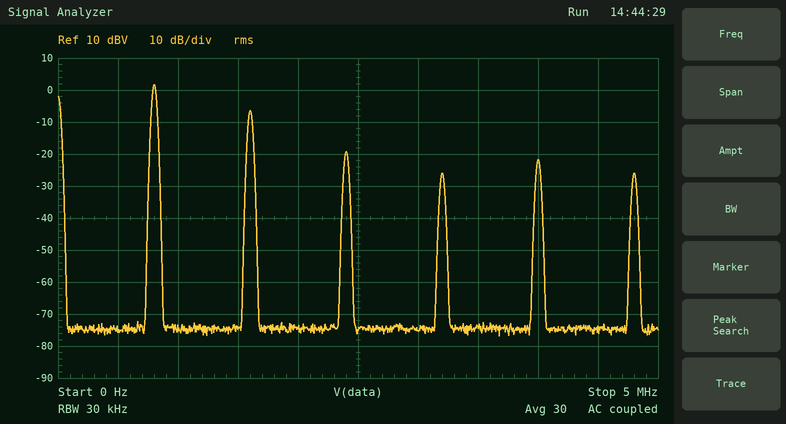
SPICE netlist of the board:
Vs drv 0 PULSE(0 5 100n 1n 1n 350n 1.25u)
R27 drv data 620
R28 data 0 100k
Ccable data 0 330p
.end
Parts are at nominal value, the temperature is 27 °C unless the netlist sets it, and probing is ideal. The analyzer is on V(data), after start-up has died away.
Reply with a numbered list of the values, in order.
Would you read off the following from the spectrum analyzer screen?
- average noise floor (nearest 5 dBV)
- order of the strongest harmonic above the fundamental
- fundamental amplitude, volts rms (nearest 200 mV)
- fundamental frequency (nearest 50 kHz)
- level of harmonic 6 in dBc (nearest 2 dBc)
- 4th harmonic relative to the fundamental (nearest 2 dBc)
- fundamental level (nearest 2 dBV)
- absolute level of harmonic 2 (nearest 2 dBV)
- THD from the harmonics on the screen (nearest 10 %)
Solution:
1. -75 dBV
2. 2
3. 1.2 V
4. 800 kHz
5. -28 dBc
6. -28 dBc
7. 2 dBV
8. -6 dBV
9. 40 %
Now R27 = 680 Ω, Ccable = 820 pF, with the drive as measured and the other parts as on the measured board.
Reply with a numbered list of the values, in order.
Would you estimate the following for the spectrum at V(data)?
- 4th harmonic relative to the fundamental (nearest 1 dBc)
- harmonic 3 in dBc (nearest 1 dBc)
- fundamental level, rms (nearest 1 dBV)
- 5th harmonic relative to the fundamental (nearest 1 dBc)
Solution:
1. -30 dBc
2. -23 dBc
3. -5 dBV
4. -26 dBc
